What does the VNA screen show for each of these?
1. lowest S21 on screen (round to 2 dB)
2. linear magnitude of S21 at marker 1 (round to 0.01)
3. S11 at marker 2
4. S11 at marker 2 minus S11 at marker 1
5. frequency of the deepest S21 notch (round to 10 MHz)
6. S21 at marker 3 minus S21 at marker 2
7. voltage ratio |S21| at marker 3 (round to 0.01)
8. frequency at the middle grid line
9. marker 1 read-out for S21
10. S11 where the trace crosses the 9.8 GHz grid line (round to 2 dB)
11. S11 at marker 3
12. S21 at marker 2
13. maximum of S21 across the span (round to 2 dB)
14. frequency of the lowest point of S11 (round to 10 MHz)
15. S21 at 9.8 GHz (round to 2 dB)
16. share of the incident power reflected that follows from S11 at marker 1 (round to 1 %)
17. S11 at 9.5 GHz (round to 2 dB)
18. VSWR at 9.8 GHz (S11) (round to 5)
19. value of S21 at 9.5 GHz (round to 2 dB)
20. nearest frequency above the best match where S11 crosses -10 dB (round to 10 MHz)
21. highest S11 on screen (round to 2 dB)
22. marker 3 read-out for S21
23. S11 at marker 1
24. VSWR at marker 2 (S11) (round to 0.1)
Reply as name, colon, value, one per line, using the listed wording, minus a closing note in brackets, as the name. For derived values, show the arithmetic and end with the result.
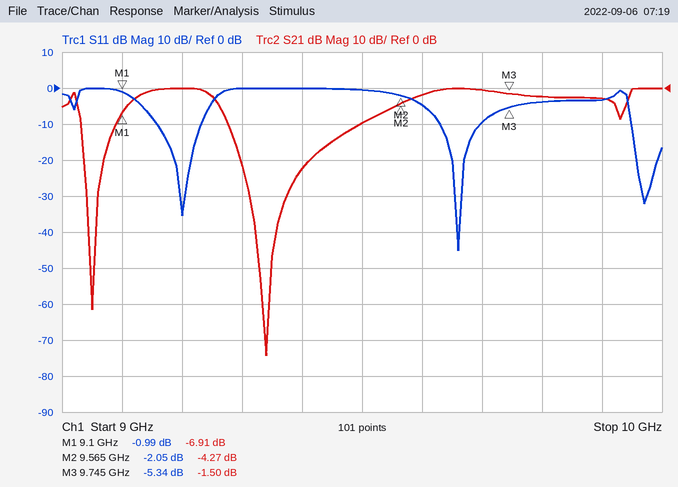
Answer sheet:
lowest S21 on screen: -74 dB
linear magnitude of S21 at marker 1: 10^(-6.91/20) ≈ 0.45
S11 at marker 2: -2.05 dB
S11 at marker 2 minus S11 at marker 1: -2.05 − (-0.99) = -1.06 dB
frequency of the deepest S21 notch: 9.34 GHz
S21 at marker 3 minus S21 at marker 2: -1.5 − (-4.27) = 2.77 dB
voltage ratio |S21| at marker 3: 10^(-1.5/20) ≈ 0.84
frequency at the middle grid line: 9.5 GHz
marker 1 read-out for S21: -6.91 dB
S11 where the trace crosses the 9.8 GHz grid line: -4 dB
S11 at marker 3: -5.34 dB
S21 at marker 2: -4.27 dB
maximum of S21 across the span: 0 dB
frequency of the lowest point of S11: 9.66 GHz
S21 at 9.8 GHz: -2 dB
share of the incident power reflected that follows from S11 at marker 1: 10^(-0.99/10) ≈ 80 %
S11 at 9.5 GHz: 0 dB
VSWR at 9.8 GHz (S11): |Γ| = 10^(-4/20) = 0.6310; VSWR = (1 + 0.6310)/(1 − 0.6310) ≈ 4.42, so 5 to the nearest 5
value of S21 at 9.5 GHz: -10 dB
nearest frequency above the best match where S11 crosses -10 dB: 9.70 GHz
highest S11 on screen: 0 dB
marker 3 read-out for S21: -1.50 dB
S11 at marker 1: -0.99 dB
VSWR at marker 2 (S11): (1 + 0.7898)/(1 − 0.7898) ≈ 8.5
